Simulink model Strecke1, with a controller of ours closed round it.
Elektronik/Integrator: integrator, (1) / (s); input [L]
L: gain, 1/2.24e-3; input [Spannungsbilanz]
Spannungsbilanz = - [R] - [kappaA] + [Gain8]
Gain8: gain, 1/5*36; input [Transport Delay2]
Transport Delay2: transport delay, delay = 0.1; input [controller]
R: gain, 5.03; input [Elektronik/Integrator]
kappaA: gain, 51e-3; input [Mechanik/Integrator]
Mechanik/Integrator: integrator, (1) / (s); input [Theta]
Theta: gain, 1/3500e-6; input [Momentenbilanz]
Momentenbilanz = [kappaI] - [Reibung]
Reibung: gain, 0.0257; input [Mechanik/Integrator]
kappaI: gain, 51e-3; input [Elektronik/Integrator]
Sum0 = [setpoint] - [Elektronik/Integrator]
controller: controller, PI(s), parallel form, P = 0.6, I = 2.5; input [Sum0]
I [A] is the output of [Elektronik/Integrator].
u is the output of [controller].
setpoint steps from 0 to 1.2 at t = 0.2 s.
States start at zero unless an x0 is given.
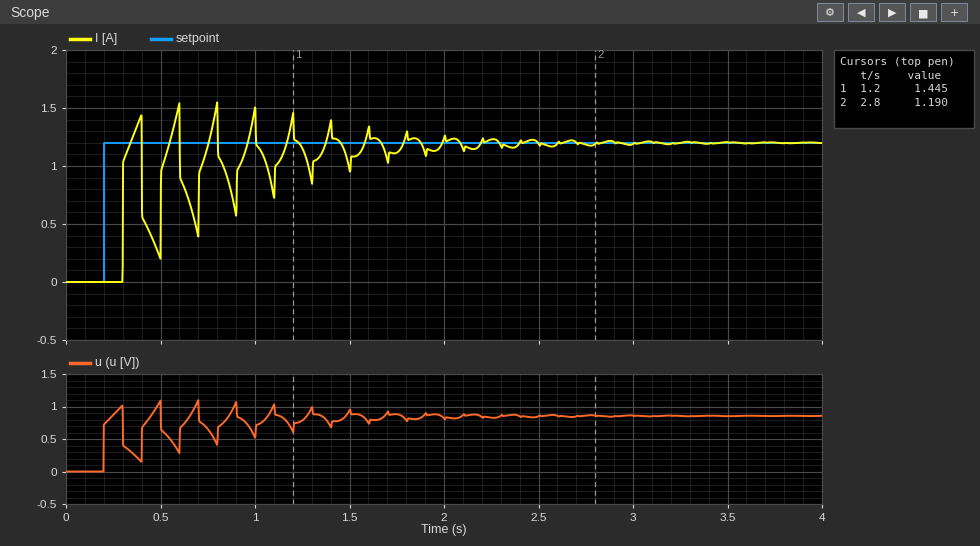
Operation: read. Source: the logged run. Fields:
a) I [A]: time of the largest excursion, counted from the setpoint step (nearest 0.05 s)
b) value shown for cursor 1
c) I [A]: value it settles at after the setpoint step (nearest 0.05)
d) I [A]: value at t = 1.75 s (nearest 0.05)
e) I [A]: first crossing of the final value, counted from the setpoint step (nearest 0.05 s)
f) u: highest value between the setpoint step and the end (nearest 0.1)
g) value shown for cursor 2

0.60 s
1.445
1.20
1.10
0.15 s
1.1
1.190
